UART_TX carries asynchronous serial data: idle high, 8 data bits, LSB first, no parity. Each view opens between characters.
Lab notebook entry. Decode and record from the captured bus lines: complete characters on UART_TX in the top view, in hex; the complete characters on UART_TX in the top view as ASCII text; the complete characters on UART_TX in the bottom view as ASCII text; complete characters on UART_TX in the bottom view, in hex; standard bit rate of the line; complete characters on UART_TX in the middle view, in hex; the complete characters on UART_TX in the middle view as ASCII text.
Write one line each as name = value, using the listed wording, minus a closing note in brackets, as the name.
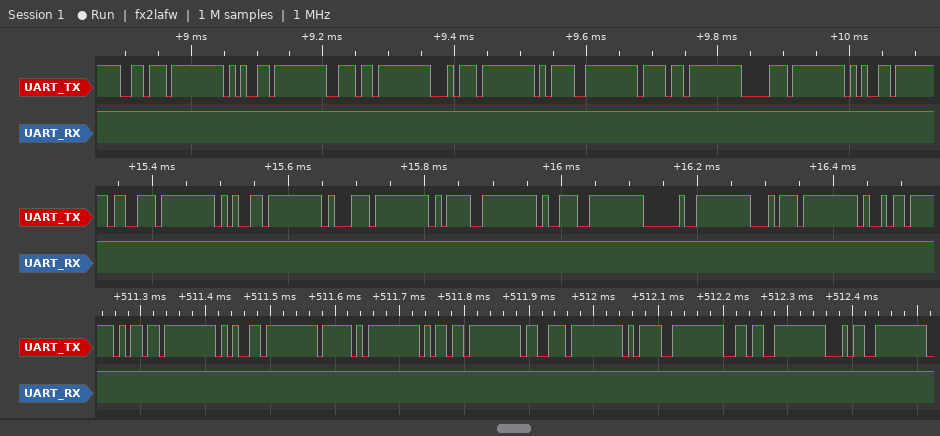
complete characters on UART_TX in the top view, in hex = 76, 65, 6E, 74, 3D, 6F, 70, 65
the complete characters on UART_TX in the top view as ASCII text = "vent=ope"
the complete characters on UART_TX in the bottom view as ASCII text = "me_ms=64"
complete characters on UART_TX in the bottom view, in hex = 6D, 65, 5F, 6D, 73, 3D, 36, 34
standard bit rate of the line = 115200 baud
complete characters on UART_TX in the middle view, in hex = 73, 65, 71, 3D, 39, 20, 74, 69
the complete characters on UART_TX in the middle view as ASCII text = "seq=9 ti"
